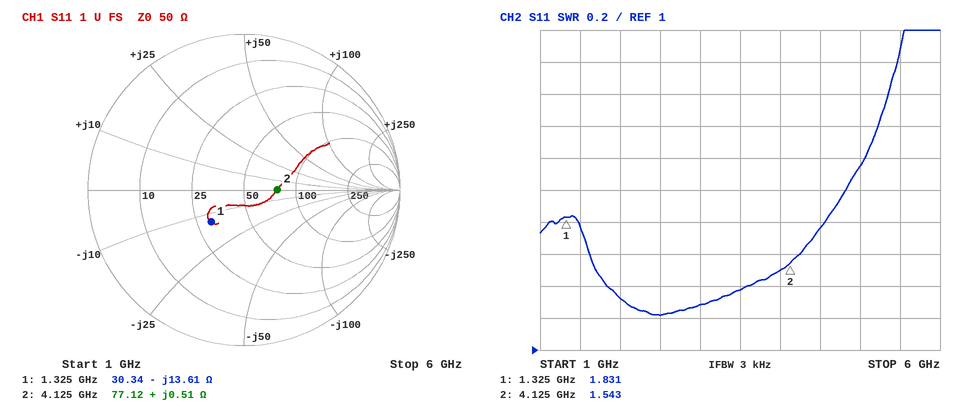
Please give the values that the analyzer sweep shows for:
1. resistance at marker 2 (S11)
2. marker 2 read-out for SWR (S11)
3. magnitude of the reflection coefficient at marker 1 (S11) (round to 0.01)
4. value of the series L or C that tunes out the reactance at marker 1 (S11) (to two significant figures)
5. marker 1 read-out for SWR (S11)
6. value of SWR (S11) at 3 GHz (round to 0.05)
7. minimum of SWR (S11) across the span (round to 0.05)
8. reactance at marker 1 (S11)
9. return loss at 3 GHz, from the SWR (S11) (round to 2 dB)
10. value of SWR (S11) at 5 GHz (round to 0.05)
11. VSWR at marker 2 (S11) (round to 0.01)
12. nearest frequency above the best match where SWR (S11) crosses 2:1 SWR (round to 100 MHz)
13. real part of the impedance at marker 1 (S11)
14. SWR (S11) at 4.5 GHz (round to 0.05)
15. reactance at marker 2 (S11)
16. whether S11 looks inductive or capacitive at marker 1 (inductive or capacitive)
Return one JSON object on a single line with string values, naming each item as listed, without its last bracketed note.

{"resistance at marker 2": "77.12 Ω", "marker 2 read-out for SWR": "1.543", "magnitude of the reflection coefficient at marker 1 (S11)": "0.29", "value of the series L or C that tunes out the reactance at marker 1 (S11)": "1.6 nH", "marker 1 read-out for SWR": "1.831", "value of SWR (S11) at 3 GHz": "1.30", "minimum of SWR (S11) across the span": "1.20", "reactance at marker 1": "-13.61 Ω", "return loss at 3 GHz, from the SWR (S11)": "18 dB", "value of SWR (S11) at 5 GHz": "2.15", "VSWR at marker 2 (S11)": "1.54", "nearest frequency above the best match where SWR (S11) crosses 2:1 SWR": "4.8 GHz", "real part of the impedance at marker 1": "30.34 Ω", "SWR (S11) at 4.5 GHz": "1.75", "reactance at marker 2": "+0.51 Ω", "whether S11 looks inductive or capacitive at marker 1": "capacitive"}
